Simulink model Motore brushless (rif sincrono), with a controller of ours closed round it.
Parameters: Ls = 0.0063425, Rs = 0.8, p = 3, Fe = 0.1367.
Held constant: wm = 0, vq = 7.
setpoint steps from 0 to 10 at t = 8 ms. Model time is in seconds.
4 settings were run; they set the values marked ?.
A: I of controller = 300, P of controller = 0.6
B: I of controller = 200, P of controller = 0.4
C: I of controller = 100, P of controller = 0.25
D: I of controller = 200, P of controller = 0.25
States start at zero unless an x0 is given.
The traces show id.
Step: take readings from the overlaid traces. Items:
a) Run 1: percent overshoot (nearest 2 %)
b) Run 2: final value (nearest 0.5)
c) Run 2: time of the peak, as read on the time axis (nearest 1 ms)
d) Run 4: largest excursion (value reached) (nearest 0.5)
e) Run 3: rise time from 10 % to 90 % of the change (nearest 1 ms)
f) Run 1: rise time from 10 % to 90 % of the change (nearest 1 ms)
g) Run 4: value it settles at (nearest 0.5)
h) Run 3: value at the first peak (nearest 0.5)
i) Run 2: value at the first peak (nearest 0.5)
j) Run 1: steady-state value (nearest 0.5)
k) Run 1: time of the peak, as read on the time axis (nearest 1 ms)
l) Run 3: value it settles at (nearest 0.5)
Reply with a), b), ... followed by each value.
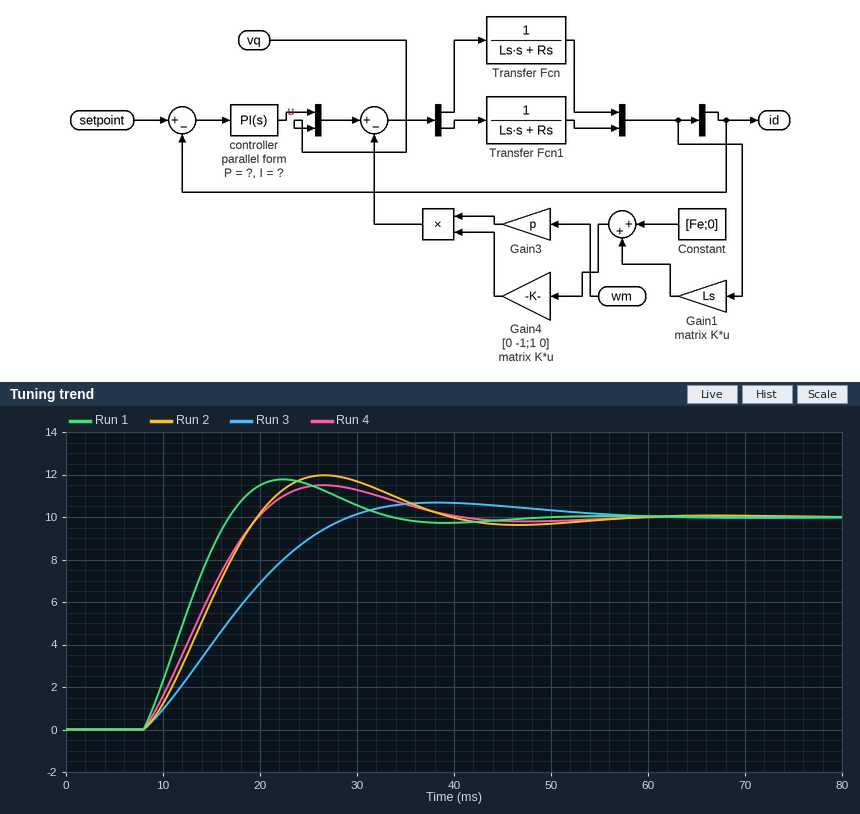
a) 18 %
b) 10.0
c) 27 ms
d) 11.5
e) 15 ms
f) 7 ms
g) 10.0
h) 10.5
i) 12.0
j) 10.0
k) 22 ms
l) 10.0
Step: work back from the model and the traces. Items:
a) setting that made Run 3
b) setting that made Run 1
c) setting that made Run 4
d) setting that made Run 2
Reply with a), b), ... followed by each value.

a) C
b) A
c) B
d) D
